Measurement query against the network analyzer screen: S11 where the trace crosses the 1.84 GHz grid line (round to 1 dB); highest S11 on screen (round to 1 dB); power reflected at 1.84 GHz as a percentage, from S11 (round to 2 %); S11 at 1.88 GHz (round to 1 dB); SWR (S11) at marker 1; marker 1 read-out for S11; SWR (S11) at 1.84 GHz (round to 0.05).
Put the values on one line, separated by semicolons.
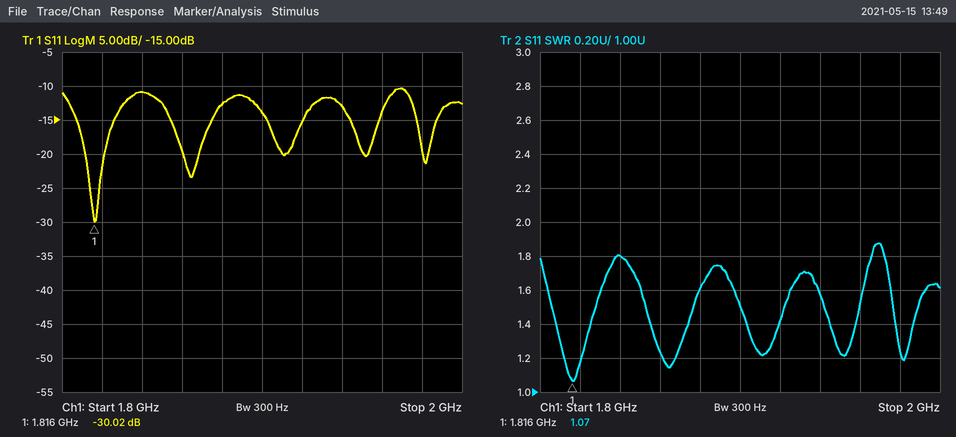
-11 dB; -10 dB; 8 %; -13 dB; 1.07; -30.02 dB; 1.80
